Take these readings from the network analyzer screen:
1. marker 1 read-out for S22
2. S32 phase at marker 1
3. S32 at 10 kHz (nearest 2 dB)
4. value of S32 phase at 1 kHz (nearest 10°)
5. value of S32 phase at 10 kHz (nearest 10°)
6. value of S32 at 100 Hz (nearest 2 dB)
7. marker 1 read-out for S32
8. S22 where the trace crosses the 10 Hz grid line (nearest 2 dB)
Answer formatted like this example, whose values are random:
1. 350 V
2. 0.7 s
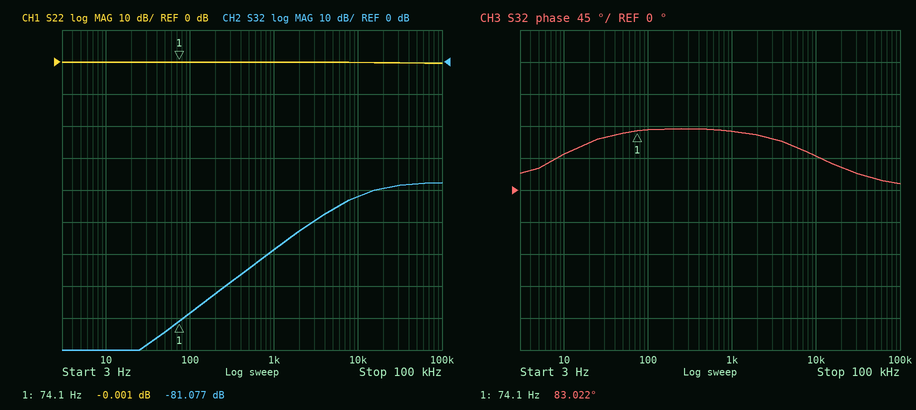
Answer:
1. -0.001 dB
2. 83.022°
3. -42 dB
4. 80°
5. 50°
6. -78 dB
7. -81.077 dB
8. 0 dB
